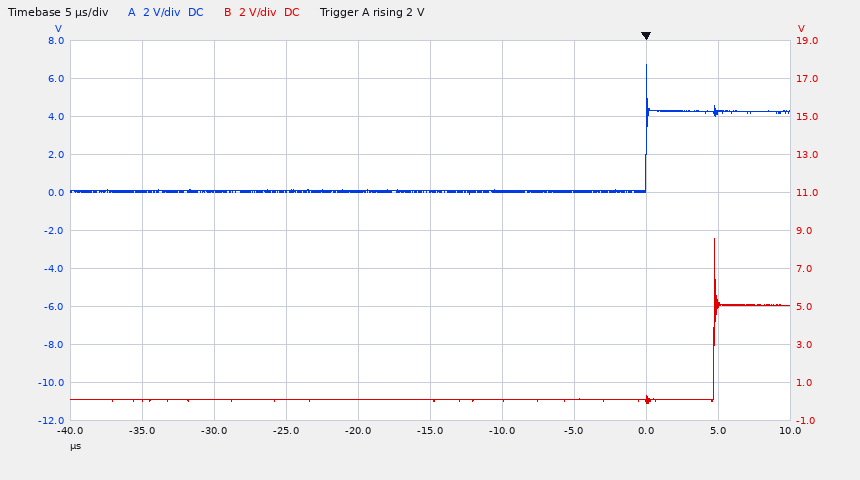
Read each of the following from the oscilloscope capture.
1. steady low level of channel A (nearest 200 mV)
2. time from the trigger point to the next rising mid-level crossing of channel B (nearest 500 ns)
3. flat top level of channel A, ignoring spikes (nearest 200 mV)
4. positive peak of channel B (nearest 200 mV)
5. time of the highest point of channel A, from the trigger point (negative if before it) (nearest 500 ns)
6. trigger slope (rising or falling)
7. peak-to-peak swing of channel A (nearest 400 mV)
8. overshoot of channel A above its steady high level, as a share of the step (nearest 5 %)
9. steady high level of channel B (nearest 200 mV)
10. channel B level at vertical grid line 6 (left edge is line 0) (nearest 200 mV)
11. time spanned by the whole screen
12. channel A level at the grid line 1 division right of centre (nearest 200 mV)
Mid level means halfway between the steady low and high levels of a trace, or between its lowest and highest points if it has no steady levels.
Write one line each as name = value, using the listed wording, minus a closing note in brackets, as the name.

steady low level of channel A = 0.0 V
time from the trigger point to the next rising mid-level crossing of channel B = 4.5 µs
flat top level of channel A, ignoring spikes = 4.2 V
positive peak of channel B = 8.6 V
time of the highest point of channel A, from the trigger point (negative if before it) = 0.0 µs
trigger slope = rising
peak-to-peak swing of channel A = 6.8 V
overshoot of channel A above its steady high level, as a share of the step = 60 %
steady high level of channel B = 5.0 V
channel B level at vertical grid line 6 (left edge is line 0) = 0.0 V
time spanned by the whole screen = 50 µs
channel A level at the grid line 1 division right of centre = 0.0 V
